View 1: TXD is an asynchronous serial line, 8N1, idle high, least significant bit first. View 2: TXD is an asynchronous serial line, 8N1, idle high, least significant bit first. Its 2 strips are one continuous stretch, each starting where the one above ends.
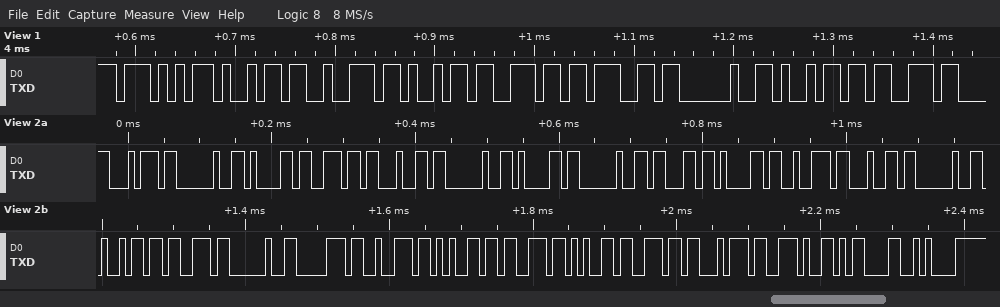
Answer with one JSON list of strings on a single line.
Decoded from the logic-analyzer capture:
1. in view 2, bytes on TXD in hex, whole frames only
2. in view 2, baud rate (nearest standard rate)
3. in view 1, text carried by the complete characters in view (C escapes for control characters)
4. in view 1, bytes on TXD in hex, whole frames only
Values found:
["74 20 61 6E 64 20 61 20 63 61 72 64 20 69 73 20 70 72 65 73 65 6E 74 2E 0D 0A", "115200 baud", "\"Wiring is\"", "57 69 72 69 6E 67 20 69 73"]
